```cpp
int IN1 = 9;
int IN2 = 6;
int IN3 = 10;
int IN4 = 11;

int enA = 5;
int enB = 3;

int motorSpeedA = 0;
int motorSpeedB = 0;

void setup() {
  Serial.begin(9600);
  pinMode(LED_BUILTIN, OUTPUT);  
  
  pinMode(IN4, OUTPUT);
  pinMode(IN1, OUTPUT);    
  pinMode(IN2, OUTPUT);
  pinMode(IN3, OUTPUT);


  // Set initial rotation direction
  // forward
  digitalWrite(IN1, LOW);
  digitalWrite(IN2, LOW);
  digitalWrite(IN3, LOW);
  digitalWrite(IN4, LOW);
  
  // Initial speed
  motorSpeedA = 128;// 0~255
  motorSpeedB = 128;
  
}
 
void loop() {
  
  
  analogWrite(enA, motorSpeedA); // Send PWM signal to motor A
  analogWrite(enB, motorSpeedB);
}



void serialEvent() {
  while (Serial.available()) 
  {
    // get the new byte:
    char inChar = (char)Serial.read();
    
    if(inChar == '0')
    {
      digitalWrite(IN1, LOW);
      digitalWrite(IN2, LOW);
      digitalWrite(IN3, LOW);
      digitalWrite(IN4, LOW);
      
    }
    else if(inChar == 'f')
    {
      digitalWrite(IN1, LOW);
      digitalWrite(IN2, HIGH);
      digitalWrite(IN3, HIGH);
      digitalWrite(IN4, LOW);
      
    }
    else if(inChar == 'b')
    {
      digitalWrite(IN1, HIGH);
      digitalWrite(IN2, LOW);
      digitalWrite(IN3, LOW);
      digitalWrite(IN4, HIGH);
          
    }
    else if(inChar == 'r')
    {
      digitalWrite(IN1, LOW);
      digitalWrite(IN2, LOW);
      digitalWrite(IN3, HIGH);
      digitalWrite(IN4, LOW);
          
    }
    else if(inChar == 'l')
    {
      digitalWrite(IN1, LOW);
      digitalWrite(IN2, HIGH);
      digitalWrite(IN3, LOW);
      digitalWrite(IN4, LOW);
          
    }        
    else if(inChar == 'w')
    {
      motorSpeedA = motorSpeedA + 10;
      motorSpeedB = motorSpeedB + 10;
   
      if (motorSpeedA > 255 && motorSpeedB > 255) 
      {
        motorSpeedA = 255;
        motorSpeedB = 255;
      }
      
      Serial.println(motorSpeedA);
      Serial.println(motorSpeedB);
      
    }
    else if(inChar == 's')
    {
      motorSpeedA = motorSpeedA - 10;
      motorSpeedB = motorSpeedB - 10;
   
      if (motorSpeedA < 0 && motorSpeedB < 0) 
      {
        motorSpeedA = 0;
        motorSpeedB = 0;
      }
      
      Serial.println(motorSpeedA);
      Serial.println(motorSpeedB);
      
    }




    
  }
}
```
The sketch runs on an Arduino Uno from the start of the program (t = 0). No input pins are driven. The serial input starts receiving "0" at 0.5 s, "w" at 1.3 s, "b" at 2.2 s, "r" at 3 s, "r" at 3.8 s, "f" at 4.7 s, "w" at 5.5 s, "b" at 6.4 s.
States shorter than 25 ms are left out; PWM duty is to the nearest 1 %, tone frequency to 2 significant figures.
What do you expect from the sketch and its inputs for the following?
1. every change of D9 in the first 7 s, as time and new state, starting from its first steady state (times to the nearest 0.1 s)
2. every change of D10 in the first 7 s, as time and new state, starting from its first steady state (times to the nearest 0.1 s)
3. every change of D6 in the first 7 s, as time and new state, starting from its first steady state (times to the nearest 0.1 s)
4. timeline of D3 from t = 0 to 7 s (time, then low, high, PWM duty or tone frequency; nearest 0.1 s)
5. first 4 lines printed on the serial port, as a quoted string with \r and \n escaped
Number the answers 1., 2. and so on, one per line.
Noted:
1. 0 s low; 2.2 s high; 3 s low; 6.4 s high
2. 0 s low; 3 s high; 6.4 s low
3. 0 s low; 4.7 s high; 6.4 s low
4. 0 s PWM 50 %; 1.3 s PWM 54 %; 5.5 s PWM 58 %
5. "138\r\n138\r\n148\r\n148\r\n"
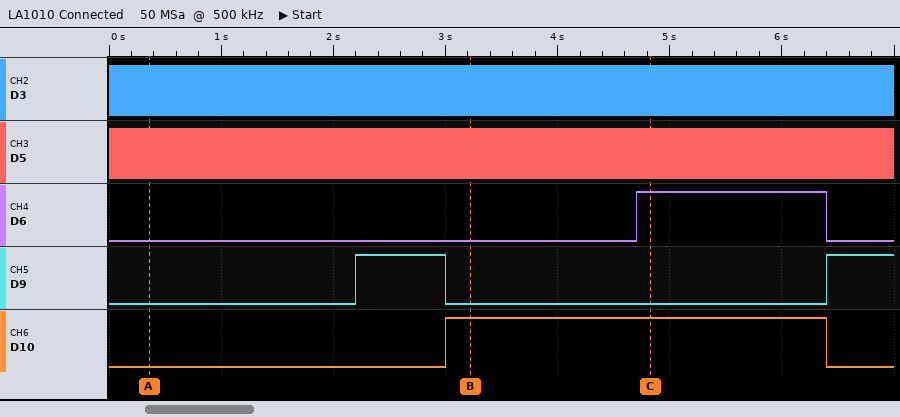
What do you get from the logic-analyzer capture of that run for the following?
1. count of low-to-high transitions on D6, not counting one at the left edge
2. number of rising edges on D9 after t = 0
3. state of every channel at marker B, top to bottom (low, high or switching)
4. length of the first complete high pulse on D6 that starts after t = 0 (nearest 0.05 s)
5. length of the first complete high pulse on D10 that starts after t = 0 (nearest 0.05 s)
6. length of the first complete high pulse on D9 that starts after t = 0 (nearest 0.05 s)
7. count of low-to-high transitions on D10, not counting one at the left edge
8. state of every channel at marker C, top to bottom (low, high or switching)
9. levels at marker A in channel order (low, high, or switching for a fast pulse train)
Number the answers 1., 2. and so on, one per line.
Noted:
1. 1
2. 2
3. D3 switching, D5 switching, D6 low, D9 low, D10 high
4. 1.70 s
5. 3.40 s
6. 0.80 s
7. 1
8. D3 switching, D5 switching, D6 high, D9 low, D10 high
9. D3 switching, D5 switching, D6 low, D9 low, D10 low
